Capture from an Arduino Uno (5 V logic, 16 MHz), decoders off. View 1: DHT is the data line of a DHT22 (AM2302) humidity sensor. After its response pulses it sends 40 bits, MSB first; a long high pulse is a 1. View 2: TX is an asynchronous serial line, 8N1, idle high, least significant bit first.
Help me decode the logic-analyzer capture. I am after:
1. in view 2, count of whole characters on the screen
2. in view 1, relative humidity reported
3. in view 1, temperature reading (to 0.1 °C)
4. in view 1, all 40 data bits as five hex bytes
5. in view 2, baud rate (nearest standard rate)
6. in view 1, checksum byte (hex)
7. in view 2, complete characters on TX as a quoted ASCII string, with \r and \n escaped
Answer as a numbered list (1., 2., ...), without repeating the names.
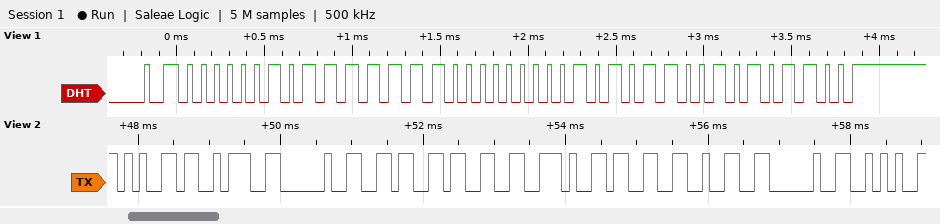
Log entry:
1. 10
2. 76.6 %
3. 17.2 °C
4. 02 FE 00 AC AC
5. 9600 baud
6. 0xAC
7. "e: 63.32 *"
